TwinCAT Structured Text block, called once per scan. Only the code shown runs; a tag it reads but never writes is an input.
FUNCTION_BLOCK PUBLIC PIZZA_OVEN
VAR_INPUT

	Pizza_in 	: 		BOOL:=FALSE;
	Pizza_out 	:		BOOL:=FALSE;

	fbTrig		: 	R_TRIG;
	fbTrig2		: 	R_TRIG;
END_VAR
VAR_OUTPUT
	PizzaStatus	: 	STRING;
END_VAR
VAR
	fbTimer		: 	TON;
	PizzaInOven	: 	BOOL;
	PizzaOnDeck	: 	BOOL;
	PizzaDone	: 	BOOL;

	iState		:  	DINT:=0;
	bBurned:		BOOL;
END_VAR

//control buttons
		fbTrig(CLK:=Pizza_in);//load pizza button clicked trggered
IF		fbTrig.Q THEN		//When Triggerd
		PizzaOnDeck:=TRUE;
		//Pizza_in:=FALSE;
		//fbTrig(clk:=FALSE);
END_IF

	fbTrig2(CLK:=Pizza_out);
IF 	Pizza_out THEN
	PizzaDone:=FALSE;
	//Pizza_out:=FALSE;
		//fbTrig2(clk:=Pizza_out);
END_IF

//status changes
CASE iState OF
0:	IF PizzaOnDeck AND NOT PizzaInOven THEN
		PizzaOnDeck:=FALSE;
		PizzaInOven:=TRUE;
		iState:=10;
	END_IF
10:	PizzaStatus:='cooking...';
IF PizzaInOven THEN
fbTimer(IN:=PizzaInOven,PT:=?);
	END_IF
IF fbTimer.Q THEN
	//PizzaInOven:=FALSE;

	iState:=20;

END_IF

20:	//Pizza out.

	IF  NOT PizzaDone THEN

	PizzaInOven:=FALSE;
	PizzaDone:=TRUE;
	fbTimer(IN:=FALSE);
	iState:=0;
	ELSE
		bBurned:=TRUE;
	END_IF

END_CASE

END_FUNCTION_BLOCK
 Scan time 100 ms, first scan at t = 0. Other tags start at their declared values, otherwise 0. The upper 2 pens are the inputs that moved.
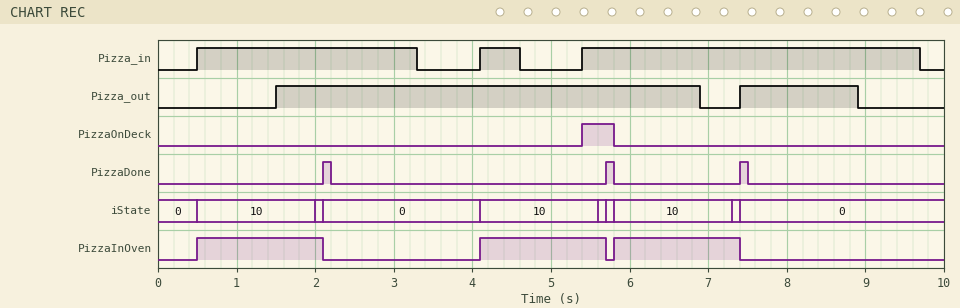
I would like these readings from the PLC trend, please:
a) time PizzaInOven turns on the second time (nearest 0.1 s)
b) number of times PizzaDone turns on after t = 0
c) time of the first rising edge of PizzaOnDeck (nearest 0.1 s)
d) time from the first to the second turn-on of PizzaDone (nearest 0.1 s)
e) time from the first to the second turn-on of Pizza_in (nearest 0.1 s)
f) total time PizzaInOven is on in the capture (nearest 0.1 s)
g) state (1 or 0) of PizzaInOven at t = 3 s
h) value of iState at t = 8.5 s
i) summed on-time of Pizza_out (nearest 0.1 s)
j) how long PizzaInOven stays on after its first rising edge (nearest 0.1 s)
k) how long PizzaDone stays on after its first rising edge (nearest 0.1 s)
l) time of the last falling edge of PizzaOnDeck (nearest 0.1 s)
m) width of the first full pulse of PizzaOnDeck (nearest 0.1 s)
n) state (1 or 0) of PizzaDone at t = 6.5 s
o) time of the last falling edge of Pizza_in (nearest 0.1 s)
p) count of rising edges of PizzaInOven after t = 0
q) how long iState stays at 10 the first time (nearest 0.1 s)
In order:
4.1 s
3
5.4 s
3.6 s
3.6 s
4.8 s
0
0
6.9 s
1.6 s
0.1 s
5.8 s
0.4 s
0
9.7 s
3
1.5 s
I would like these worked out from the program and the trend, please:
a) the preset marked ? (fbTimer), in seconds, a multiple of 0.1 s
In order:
1.4 s
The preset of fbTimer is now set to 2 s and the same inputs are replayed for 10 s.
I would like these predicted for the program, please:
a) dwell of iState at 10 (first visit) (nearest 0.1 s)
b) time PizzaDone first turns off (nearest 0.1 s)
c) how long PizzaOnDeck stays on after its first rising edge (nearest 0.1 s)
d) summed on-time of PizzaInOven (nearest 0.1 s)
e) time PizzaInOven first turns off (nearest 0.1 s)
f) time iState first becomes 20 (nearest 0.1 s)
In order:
2.1 s
2.8 s
1.0 s
6.6 s
2.7 s
2.6 s
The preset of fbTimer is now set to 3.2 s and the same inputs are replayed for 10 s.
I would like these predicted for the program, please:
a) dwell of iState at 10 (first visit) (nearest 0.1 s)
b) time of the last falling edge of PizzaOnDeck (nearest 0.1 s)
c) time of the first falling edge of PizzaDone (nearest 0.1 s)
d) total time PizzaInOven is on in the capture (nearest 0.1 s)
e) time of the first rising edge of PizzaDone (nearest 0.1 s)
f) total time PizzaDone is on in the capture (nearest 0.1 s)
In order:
3.3 s
7.6 s
4.0 s
9.2 s
3.9 s
0.2 s
